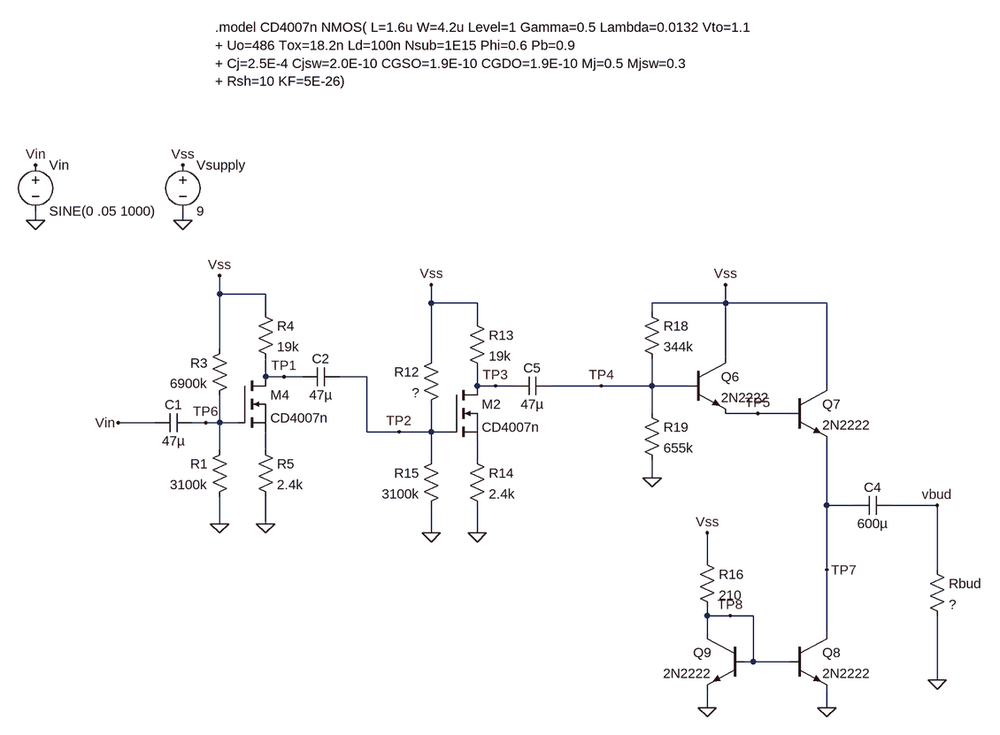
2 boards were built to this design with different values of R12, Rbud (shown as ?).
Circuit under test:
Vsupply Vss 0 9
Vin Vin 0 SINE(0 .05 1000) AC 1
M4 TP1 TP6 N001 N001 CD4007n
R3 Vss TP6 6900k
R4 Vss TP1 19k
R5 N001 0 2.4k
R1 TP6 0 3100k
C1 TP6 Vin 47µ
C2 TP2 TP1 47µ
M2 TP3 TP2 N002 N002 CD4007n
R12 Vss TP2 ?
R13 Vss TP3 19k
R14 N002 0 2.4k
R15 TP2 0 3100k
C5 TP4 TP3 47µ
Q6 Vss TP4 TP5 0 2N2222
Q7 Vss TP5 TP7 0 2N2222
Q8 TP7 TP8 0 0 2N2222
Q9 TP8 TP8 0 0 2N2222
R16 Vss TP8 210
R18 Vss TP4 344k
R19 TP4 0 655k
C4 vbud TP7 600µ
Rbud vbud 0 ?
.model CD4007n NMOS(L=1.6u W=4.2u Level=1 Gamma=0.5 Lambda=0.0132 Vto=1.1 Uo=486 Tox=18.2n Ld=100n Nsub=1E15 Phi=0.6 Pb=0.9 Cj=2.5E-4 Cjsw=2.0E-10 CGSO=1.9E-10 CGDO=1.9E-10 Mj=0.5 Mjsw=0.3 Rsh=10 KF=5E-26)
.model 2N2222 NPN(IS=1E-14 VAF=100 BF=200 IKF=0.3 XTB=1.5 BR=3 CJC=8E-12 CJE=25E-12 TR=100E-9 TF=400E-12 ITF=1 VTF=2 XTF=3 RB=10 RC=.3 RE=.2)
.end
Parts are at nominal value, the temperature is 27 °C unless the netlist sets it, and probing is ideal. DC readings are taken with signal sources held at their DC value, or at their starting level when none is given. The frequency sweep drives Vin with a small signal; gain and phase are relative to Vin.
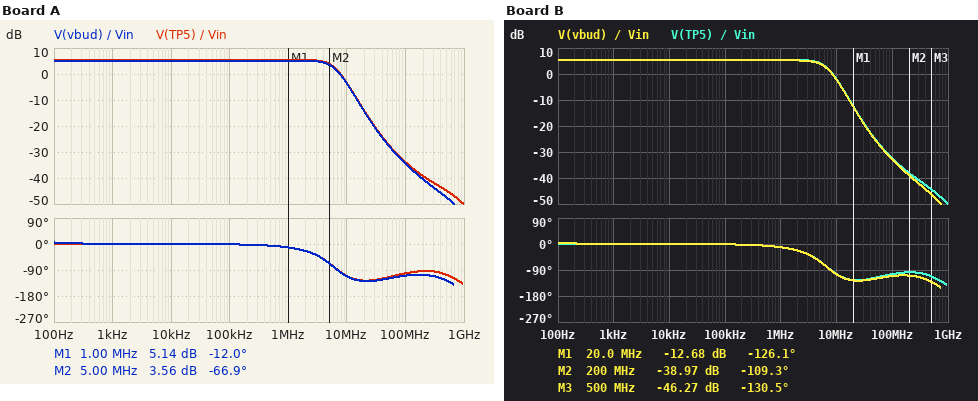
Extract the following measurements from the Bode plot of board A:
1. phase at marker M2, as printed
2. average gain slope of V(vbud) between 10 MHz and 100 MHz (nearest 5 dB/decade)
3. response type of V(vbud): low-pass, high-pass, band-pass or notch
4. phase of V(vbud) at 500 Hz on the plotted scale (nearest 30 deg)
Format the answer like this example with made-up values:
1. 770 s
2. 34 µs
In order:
1. -66.9 deg
2. -30 dB/decade
3. low-pass
4. 0 deg
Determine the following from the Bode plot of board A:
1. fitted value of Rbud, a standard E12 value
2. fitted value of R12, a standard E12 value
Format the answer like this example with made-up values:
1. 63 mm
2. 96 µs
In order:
1. 27 Ω
2. 3.9 MΩ
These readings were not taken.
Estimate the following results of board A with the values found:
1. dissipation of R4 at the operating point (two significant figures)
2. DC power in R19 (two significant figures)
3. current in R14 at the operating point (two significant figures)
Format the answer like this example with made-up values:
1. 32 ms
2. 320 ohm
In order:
1. 820 µW
2. 49 µW
3. 380 µA
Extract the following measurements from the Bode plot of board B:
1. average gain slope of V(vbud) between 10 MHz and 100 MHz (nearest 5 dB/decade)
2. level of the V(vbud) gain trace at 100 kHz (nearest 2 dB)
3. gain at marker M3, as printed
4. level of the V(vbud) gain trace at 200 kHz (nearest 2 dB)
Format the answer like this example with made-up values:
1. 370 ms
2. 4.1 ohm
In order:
1. -30 dB/decade
2. 6 dB
3. -46.27 dB
4. 6 dB
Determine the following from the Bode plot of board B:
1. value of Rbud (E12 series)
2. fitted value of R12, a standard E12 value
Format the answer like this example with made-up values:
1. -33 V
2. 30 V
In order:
1. 39 Ω
2. 3.9 MΩ
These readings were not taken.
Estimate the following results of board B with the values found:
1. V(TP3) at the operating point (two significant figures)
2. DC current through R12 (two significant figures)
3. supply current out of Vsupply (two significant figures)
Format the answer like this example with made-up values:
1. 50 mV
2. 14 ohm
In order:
1. 1.8 V
2. 1.3 µA
3. 80 mA
